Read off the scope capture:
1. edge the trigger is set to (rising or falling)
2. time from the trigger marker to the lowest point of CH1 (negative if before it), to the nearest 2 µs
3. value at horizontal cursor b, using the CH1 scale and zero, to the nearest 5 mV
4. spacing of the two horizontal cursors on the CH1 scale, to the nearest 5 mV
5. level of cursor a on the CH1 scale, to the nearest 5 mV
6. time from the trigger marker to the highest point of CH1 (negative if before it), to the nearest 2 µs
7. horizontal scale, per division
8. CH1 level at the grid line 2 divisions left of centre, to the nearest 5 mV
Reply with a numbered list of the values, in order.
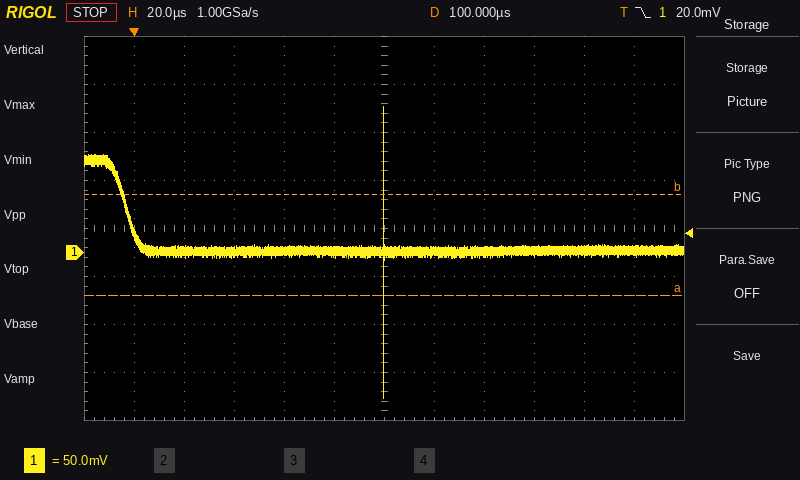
1. falling
2. +100 µs
3. 60 mV
4. 105 mV
5. -45 mV
6. +100 µs
7. 20 µs
8. 0 mV
